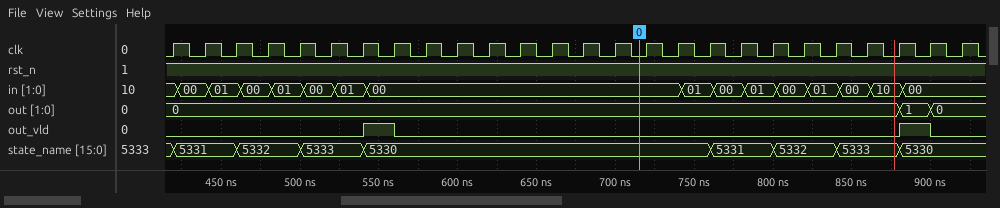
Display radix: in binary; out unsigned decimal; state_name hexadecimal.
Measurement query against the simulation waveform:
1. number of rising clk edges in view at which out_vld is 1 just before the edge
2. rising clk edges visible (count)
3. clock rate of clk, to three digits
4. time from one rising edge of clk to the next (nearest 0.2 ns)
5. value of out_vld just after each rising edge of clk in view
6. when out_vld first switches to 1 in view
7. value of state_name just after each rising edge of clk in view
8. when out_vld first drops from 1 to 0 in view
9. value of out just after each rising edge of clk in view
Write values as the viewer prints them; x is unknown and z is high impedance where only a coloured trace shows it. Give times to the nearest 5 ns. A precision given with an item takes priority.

2
26
50.0 MHz
20 ns
0 0 0 0 0 0 1 0 0 0 0 0 0 0 0 0 0 0 0 0 0 0 0 1 0 0
540 ns
5331, 5331, 5332, 5332, 5333, 5333, 5330, 5330, 5330, 5330, 5330, 5330, 5330, 5330, 5330, 5330, 5330, 5331, 5331, 5332, 5332, 5333, 5333, 5330, 5330, 5330
560 ns
0, 0, 0, 0, 0, 0, 0, 0, 0, 0, 0, 0, 0, 0, 0, 0, 0, 0, 0, 0, 0, 0, 0, 1, 0, 0
